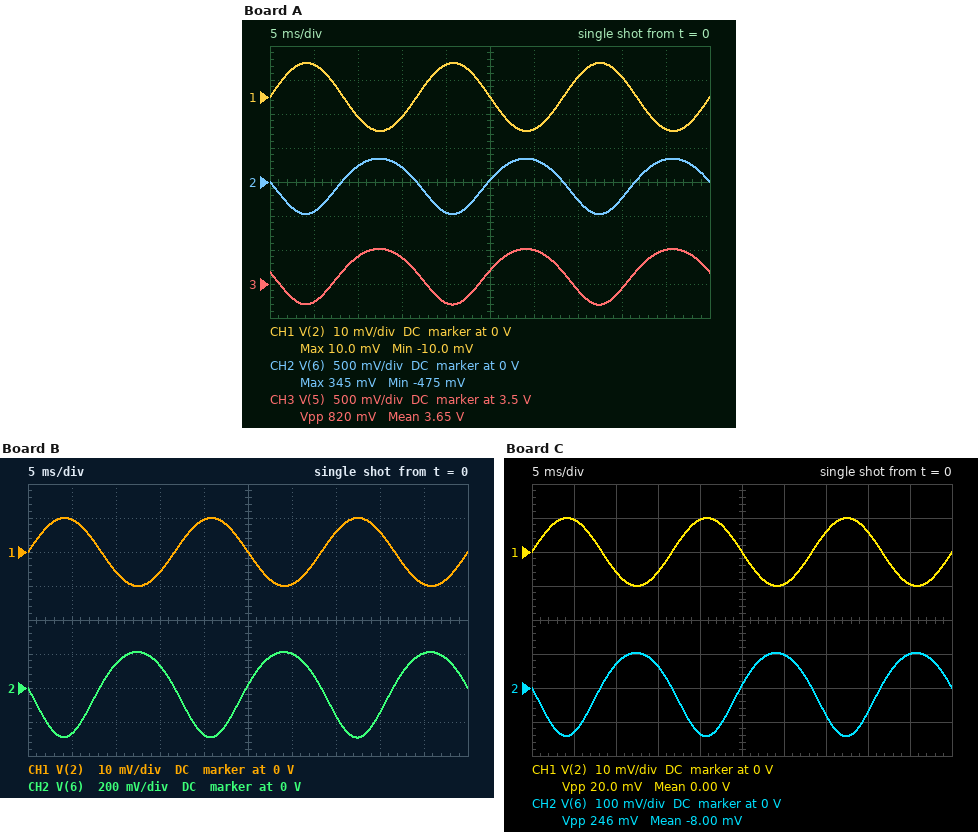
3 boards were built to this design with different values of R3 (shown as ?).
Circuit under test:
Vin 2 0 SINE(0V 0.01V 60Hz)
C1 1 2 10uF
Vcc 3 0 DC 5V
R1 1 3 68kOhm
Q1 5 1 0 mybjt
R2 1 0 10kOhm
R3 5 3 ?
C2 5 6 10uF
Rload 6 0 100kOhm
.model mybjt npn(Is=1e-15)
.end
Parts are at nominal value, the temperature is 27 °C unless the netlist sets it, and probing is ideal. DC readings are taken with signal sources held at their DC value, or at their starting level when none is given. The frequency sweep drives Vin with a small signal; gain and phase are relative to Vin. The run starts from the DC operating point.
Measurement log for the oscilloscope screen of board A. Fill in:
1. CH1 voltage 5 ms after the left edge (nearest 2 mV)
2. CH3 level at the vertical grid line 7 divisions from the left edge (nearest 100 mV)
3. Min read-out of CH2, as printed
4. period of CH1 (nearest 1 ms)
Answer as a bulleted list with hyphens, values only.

- 10 mV
- 3.4 V
- -475 mV
- 17 ms
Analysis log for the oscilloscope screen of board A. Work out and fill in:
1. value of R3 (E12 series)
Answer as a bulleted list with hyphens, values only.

- 27 kΩ
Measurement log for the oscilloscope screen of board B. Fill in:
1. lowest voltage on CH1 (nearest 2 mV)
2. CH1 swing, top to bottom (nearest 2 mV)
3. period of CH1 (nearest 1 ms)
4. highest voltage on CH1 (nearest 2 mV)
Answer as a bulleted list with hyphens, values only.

- -10 mV
- 20 mV
- 17 ms
- 10 mV
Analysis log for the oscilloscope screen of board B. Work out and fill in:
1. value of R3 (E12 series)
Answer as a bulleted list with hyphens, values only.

- 15 kΩ
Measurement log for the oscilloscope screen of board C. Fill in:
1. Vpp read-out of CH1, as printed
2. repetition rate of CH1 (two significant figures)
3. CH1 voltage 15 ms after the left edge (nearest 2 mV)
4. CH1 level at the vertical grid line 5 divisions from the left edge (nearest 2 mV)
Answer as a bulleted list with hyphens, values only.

- 20.0 mV
- 60 Hz
- -6 mV
- 0 V
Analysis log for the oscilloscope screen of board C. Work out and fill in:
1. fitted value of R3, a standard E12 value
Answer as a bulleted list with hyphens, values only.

- 6.8 kΩ
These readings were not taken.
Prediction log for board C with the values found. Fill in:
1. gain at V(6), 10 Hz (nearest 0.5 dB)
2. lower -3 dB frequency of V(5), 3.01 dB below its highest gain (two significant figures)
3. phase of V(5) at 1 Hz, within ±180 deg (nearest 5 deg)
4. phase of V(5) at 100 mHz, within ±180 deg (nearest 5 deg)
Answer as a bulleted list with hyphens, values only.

- 21.5 dB
- 2.1 Hz
- -115 deg
- -95 deg
